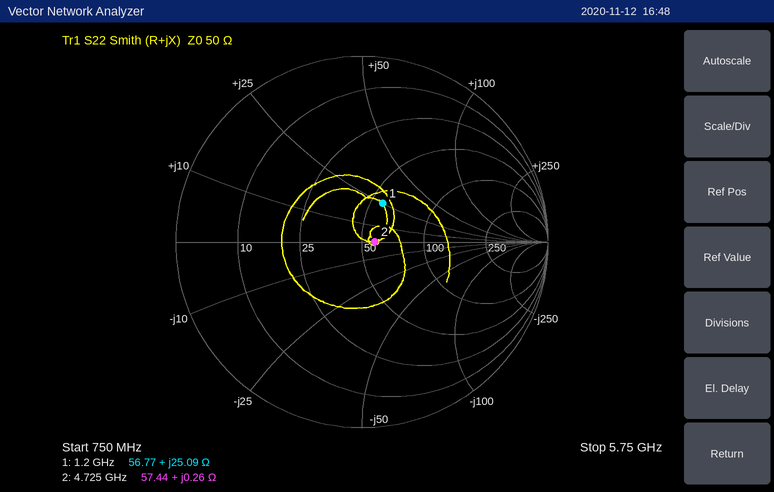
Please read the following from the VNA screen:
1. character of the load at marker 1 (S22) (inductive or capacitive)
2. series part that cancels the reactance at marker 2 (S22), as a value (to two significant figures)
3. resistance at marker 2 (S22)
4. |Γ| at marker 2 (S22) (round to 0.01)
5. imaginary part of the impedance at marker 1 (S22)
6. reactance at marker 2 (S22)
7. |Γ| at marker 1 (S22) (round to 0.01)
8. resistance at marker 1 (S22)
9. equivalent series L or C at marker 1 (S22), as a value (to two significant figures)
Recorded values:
inductive
130 pF
57.44 Ω
0.07
+25.09 Ω
+0.26 Ω
0.24
56.77 Ω
3.3 nH
